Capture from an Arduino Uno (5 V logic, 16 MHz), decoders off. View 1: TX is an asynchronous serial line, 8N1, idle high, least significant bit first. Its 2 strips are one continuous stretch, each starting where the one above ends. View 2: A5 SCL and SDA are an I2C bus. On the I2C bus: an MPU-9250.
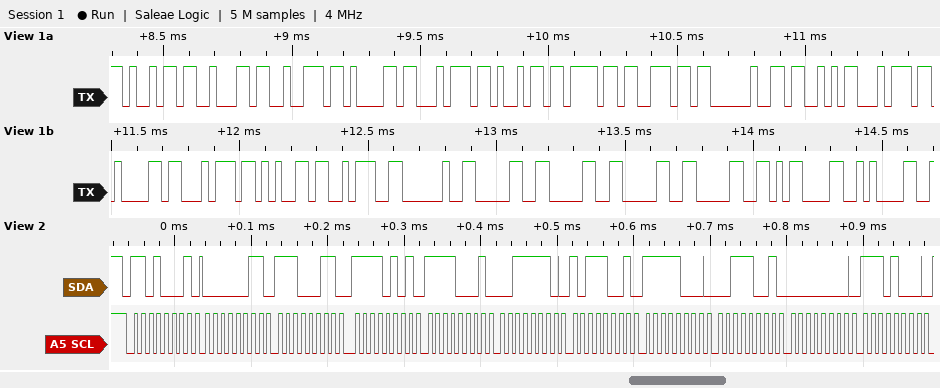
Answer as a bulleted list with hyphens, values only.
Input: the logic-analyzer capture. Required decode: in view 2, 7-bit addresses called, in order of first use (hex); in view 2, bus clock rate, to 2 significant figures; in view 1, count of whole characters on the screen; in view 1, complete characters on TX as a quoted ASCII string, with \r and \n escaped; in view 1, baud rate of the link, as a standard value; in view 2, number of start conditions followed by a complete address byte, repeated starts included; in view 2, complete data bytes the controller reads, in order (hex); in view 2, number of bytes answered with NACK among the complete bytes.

- 0x68
- 100 kHz
- 22
- "ibration State: 0000\r\n"
- 38400 baud
- 1
- 03 E3 F5 F1 3E B9 F8 39 00 E8
- 0
